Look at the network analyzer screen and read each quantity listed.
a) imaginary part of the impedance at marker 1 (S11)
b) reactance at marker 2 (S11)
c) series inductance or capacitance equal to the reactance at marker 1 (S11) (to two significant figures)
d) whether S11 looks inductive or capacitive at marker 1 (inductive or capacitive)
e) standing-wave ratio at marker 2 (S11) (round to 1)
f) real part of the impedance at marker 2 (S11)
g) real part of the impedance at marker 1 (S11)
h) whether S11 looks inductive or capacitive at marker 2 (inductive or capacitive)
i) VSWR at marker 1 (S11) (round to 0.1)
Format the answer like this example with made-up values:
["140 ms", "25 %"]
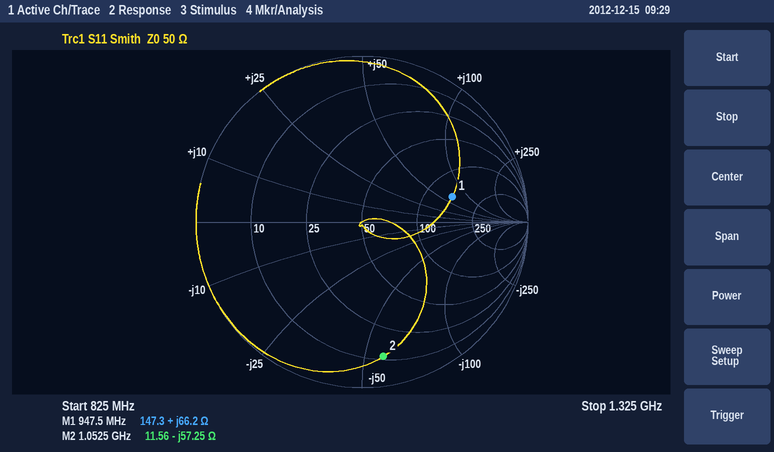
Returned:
["+66.2 Ω", "-57.25 Ω", "11 nH", "inductive", "10", "11.56 Ω", "147.3 Ω", "capacitive", "3.6"]
